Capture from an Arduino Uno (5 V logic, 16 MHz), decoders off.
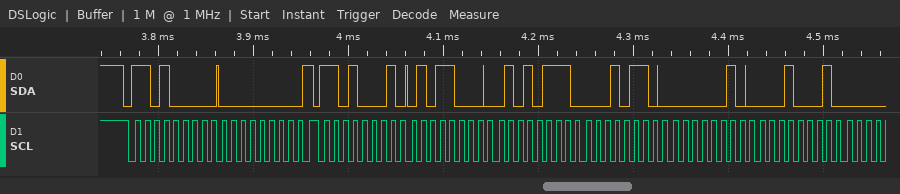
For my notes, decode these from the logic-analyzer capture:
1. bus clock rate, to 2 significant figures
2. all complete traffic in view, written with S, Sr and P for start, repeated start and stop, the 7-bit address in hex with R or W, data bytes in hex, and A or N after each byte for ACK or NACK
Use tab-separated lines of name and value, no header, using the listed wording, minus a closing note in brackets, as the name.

bus clock rate, to 2 significant figures	100 kHz
all complete traffic in view, written with S, Sr and P for start, repeated start and stop, the 7-bit address in hex with R or W, data bytes in hex, and A or N after each byte for ACK or NACK	S 68W A 00 A Sr 68R A 58 A 57 A 16 A 02 A 11 A
